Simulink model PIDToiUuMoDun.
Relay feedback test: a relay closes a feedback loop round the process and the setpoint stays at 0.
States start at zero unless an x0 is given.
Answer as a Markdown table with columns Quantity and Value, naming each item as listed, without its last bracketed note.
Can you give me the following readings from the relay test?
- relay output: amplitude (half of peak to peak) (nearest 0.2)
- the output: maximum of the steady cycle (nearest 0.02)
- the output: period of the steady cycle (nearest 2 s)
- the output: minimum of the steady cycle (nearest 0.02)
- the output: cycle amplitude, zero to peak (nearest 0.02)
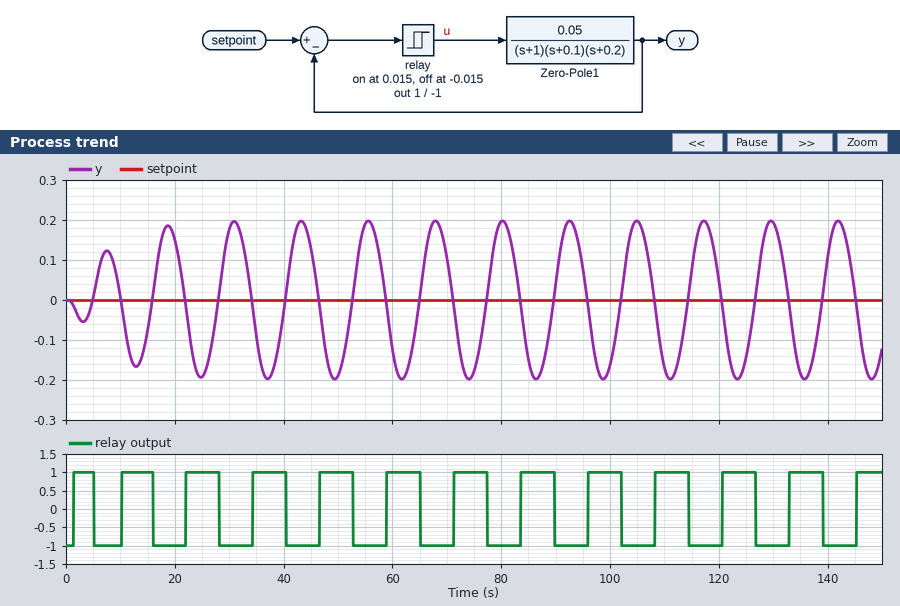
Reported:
| Quantity | Value |
|---|---|
| relay output: amplitude (half of peak to peak) | 1.0 |
| the output: maximum of the steady cycle | 0.20 |
| the output: period of the steady cycle | 12 s |
| the output: minimum of the steady cycle | -0.20 |
| the output: cycle amplitude, zero to peak | 0.20 |
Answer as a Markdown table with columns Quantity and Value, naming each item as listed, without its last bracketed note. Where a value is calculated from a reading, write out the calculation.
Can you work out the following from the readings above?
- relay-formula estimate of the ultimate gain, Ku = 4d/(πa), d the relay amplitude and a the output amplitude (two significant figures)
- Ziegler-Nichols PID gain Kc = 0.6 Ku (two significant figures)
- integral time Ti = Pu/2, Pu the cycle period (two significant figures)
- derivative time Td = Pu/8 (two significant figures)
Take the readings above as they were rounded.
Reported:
| Quantity | Value |
|---|---|
| relay-formula estimate of the ultimate gain, Ku = 4d/(πa), d the relay amplitude and a the output amplitude | 4 × 1 / (π × 0.2) = 6.4 |
| Ziegler-Nichols PID gain Kc = 0.6 Ku | 0.6 × 6.4 = 3.8 |
| integral time Ti = Pu/2, Pu the cycle period | 12 / 2 = 6.0 s |
| derivative time Td = Pu/8 | 12 / 8 = 1.5 s |
